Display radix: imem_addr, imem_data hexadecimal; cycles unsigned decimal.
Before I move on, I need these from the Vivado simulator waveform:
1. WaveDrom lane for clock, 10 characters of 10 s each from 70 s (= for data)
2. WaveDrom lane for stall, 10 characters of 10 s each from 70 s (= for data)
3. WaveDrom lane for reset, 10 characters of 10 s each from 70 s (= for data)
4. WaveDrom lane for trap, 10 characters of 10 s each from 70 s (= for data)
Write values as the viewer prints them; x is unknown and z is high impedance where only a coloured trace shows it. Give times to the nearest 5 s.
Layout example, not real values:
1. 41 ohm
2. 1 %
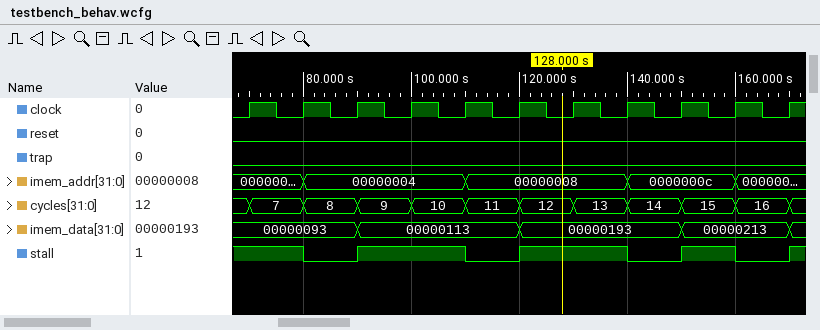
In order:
1. {name: 'clock', wave: 'p.........'}
2. {name: 'stall', wave: '101.01.010'}
3. {name: 'reset', wave: '0.........'}
4. {name: 'trap', wave: '0.........'}
